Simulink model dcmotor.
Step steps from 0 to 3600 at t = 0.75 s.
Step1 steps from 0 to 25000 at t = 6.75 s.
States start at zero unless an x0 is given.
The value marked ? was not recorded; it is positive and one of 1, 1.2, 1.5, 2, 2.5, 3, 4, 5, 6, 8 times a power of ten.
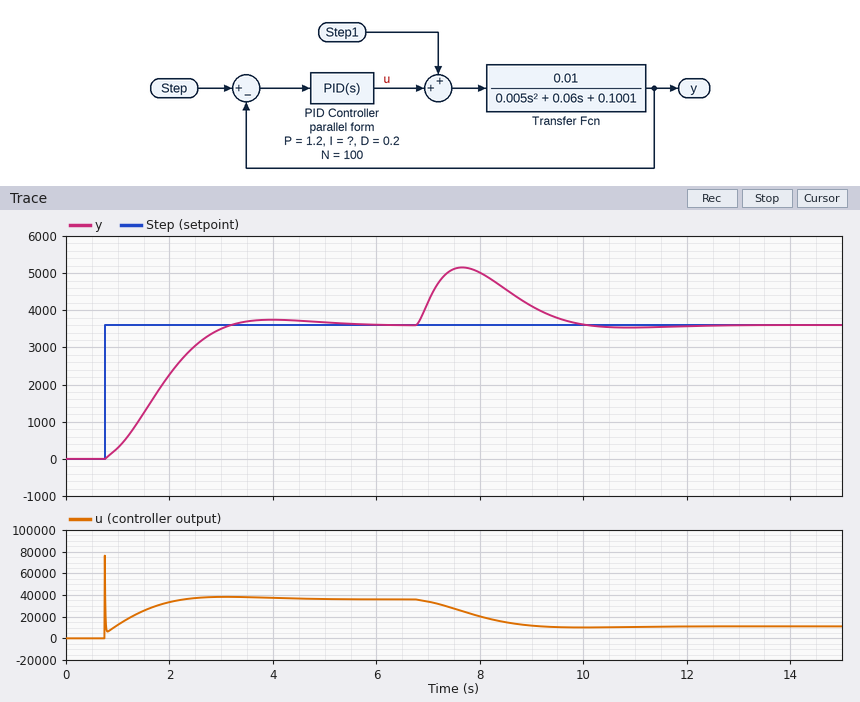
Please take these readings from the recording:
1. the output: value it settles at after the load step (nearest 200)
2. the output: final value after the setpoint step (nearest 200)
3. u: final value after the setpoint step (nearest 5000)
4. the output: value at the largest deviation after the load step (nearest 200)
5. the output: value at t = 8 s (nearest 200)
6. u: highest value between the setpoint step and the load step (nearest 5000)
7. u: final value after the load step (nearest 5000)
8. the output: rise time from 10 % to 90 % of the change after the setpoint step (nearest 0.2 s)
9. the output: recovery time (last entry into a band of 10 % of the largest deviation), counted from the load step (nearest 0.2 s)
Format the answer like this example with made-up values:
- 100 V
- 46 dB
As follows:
- 3600
- 3600
- 35000
- 5200
- 5000
- 75000
- 10000
- 1.6 s
- 2.8 s
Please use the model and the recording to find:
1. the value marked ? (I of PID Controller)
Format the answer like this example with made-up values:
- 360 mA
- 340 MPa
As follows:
- 10
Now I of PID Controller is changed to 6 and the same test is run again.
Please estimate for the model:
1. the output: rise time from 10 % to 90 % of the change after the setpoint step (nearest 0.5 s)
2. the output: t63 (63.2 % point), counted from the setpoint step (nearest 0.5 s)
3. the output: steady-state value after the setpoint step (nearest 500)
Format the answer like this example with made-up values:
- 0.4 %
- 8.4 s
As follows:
- 3.0 s
- 2.0 s
- 3500
